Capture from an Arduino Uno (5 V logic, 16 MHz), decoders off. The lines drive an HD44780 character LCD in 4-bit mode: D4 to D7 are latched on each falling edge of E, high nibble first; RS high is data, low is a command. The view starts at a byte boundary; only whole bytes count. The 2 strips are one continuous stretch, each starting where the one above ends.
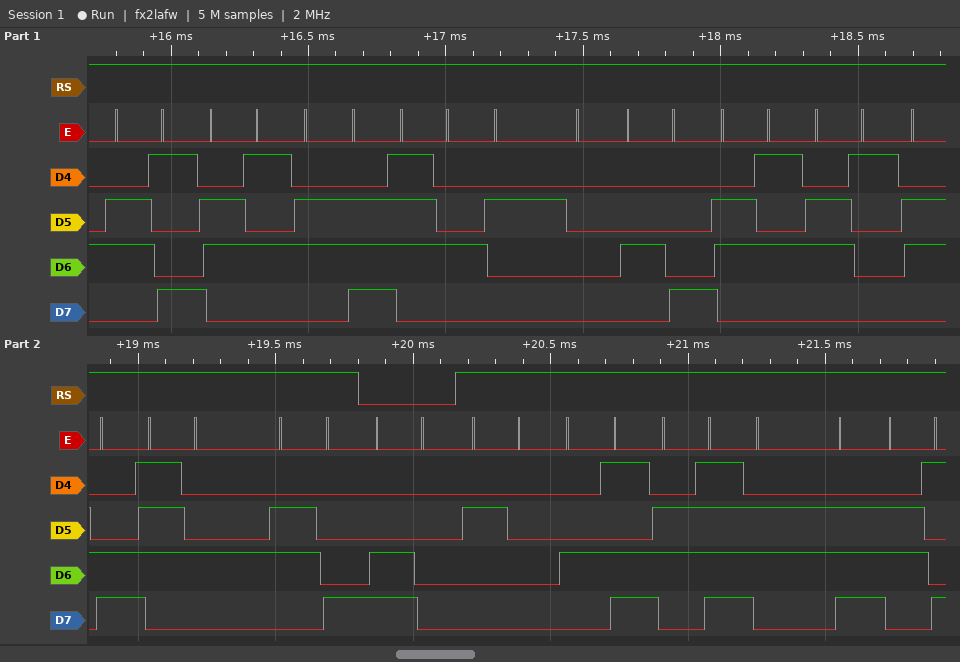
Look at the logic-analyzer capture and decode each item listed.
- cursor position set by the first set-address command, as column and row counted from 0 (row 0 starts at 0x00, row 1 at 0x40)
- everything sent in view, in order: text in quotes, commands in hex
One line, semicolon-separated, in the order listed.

column 0, row 1; "ient Health" 0xC0 " Moni"
